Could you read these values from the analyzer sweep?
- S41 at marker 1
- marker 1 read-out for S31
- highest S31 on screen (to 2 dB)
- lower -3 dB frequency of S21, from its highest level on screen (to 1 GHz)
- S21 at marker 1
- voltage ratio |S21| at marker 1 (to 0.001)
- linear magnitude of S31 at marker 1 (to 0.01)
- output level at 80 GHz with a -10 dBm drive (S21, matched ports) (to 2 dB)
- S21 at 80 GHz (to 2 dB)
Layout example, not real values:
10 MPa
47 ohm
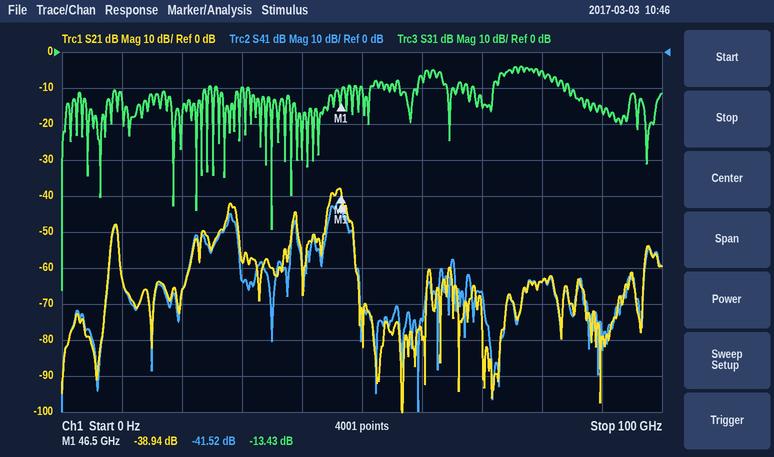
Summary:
-41.52 dB
-13.43 dB
-4 dB
45 GHz
-38.94 dB
0.011
0.21
-74 dBm
-64 dB
